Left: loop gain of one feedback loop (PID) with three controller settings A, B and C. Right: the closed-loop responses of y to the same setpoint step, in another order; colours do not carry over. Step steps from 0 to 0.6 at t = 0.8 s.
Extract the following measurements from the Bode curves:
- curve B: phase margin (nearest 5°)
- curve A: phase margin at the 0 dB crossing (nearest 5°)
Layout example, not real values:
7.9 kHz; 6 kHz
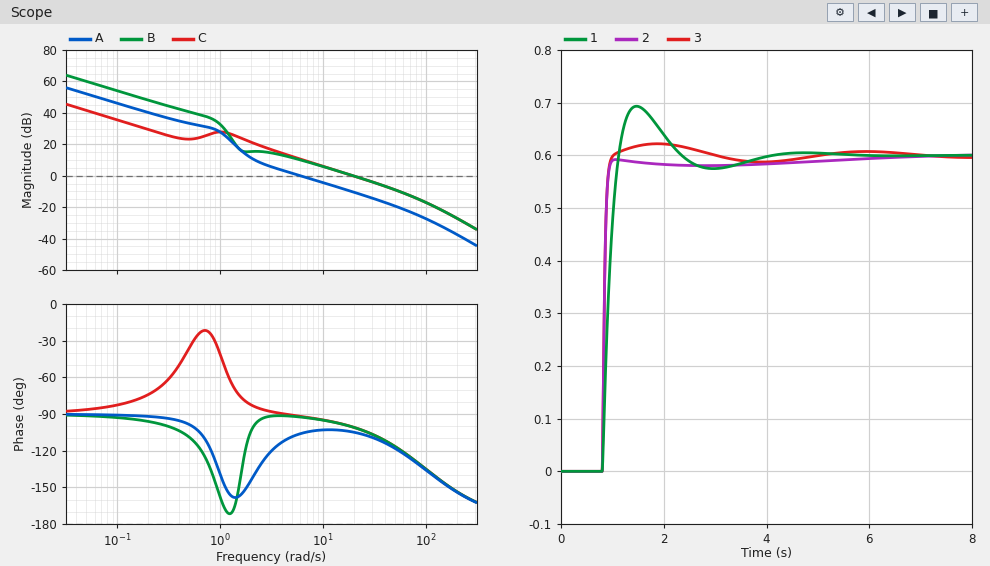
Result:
80°; 75°
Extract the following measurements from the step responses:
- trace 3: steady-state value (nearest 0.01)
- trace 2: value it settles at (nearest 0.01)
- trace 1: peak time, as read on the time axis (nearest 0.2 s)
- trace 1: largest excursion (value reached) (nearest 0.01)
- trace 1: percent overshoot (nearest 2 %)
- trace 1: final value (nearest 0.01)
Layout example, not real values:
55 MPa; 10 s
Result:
0.60; 0.60; 1.4 s; 0.69; 16 %; 0.60
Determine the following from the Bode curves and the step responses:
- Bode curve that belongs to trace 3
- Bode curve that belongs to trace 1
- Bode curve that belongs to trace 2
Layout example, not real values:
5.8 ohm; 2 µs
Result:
B; A; C
